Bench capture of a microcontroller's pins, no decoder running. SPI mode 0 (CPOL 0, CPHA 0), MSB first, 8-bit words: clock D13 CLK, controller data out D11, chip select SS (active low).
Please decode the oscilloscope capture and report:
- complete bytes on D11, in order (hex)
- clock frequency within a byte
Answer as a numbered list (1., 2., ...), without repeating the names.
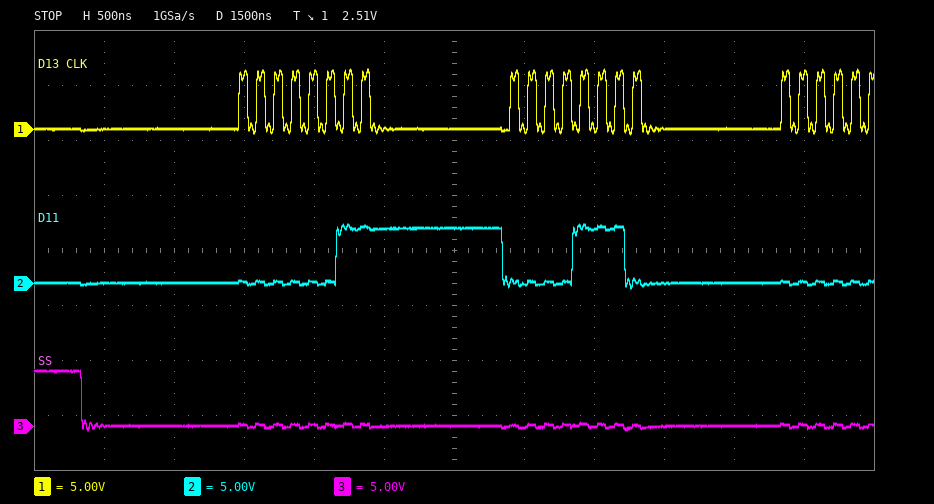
1. 03 0E
2. 8 MHz
